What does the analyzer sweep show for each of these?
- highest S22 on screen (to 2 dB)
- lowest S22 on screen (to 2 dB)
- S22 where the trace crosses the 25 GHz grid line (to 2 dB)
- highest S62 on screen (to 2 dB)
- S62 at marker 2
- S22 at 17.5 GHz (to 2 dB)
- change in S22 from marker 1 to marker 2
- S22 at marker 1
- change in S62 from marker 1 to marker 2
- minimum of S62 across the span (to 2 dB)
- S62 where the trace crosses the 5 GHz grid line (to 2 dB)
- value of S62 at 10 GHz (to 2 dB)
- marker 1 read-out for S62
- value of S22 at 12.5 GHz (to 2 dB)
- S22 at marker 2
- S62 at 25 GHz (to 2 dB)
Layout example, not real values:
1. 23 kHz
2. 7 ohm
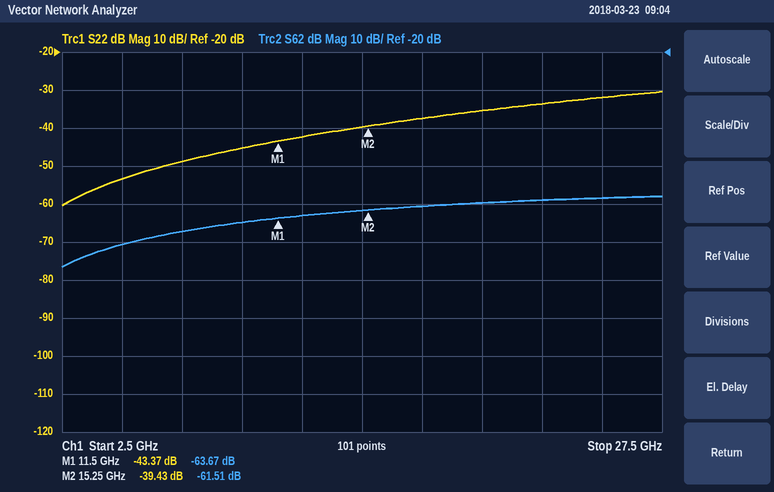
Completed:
1. -30 dB
2. -60 dB
3. -32 dB
4. -58 dB
5. -61.51 dB
6. -38 dB
7. 3.94 dB
8. -43.37 dB
9. 2.16 dB
10. -76 dB
11. -70 dB
12. -64 dB
13. -63.67 dB
14. -42 dB
15. -39.43 dB
16. -58 dB
